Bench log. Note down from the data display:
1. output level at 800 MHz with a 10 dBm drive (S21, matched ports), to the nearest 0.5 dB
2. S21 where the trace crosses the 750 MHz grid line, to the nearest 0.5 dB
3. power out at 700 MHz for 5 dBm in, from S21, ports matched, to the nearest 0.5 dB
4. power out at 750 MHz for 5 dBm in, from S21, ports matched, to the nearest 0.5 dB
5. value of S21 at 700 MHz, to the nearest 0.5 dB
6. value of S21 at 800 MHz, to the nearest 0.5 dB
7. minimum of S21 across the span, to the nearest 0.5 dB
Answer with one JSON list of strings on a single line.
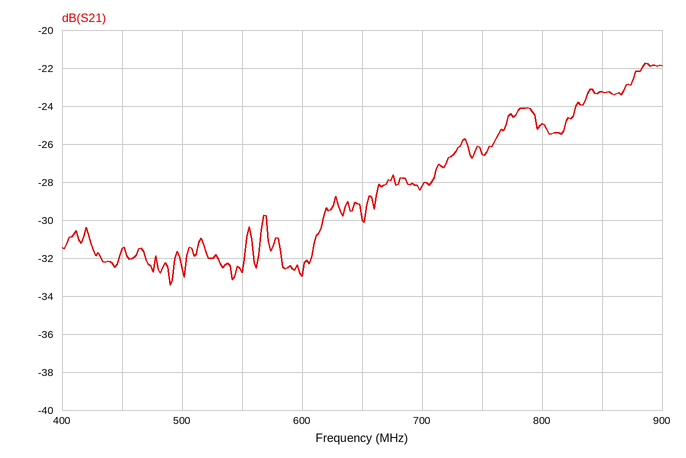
["-15.0 dBm", "-26.5 dB", "-23.0 dBm", "-21.5 dBm", "-28.0 dB", "-25.0 dB", "-33.5 dB"]
